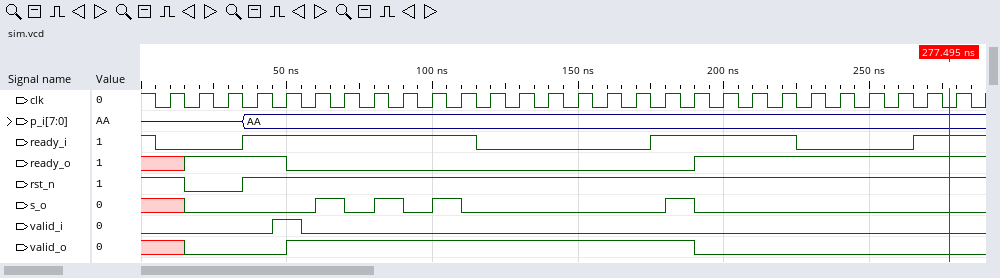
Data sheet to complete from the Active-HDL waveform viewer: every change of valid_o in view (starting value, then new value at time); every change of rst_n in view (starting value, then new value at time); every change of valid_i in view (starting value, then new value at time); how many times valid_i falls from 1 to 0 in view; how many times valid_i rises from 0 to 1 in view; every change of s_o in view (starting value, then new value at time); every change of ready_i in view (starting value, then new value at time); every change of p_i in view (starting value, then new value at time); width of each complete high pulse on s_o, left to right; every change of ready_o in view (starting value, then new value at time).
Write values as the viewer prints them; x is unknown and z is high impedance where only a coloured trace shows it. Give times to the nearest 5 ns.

x, 0 at 15 ns, 1 at 50 ns, 0 at 190 ns
1, 0 at 15 ns, 1 at 35 ns
0, 1 at 45 ns, 0 at 55 ns
1
1
x, 0 at 15 ns, 1 at 60 ns, 0 at 70 ns, 1 at 80 ns, 0 at 90 ns, 1 at 100 ns, 0 at 110 ns, 1 at 180 ns, 0 at 190 ns
1, 0 at 5 ns, 1 at 35 ns, 0 at 115 ns, 1 at 175 ns, 0 at 225 ns, 1 at 265 ns
z, AA at 35 ns
10 ns, 10 ns, 10 ns, 10 ns
x, 1 at 15 ns, 0 at 50 ns, 1 at 190 ns
